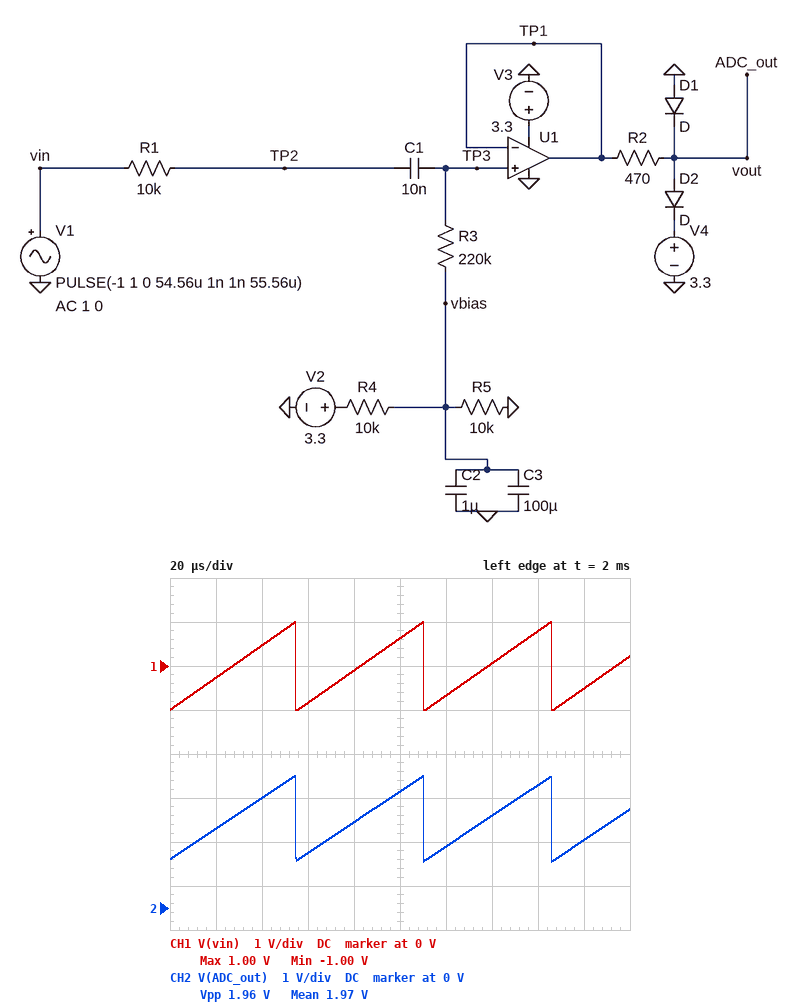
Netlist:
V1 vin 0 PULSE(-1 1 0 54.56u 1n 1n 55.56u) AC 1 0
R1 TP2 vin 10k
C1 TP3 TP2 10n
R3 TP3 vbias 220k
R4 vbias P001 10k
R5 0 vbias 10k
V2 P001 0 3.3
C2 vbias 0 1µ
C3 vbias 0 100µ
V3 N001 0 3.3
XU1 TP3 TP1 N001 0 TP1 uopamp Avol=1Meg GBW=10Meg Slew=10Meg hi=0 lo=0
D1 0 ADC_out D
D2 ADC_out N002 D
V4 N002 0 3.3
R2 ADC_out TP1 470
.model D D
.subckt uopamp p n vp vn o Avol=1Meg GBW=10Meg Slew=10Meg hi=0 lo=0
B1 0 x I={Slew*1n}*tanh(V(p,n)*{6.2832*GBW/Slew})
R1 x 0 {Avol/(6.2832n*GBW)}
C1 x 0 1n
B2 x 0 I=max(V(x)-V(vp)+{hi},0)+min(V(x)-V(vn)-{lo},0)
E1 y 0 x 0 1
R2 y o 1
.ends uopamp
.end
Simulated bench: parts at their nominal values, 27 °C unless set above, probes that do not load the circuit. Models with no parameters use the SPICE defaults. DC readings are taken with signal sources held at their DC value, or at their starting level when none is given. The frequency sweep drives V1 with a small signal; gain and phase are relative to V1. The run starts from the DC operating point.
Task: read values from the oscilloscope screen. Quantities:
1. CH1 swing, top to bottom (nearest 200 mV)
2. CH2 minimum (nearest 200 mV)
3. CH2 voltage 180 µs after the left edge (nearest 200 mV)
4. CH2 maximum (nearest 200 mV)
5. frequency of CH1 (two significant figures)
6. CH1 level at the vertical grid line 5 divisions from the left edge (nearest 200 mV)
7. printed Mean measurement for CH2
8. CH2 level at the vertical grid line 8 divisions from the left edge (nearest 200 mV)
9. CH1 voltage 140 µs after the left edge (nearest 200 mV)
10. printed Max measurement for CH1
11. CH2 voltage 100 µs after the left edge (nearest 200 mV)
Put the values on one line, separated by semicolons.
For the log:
2.0 V; 1.0 V; 1.6 V; 3.0 V; 18 kHz; 600 mV; 1.97 V; 2.8 V; 0 V; 1.00 V; 2.6 V
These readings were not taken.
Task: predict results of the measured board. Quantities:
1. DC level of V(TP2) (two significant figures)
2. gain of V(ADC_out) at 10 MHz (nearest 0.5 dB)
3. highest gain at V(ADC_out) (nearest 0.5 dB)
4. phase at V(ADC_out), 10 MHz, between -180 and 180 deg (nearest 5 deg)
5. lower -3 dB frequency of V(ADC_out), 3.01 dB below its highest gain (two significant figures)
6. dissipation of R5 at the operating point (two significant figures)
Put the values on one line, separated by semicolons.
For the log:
-1.0 V; -3.5 dB; -0.5 dB; -45 deg; 69 Hz; 270 µW
